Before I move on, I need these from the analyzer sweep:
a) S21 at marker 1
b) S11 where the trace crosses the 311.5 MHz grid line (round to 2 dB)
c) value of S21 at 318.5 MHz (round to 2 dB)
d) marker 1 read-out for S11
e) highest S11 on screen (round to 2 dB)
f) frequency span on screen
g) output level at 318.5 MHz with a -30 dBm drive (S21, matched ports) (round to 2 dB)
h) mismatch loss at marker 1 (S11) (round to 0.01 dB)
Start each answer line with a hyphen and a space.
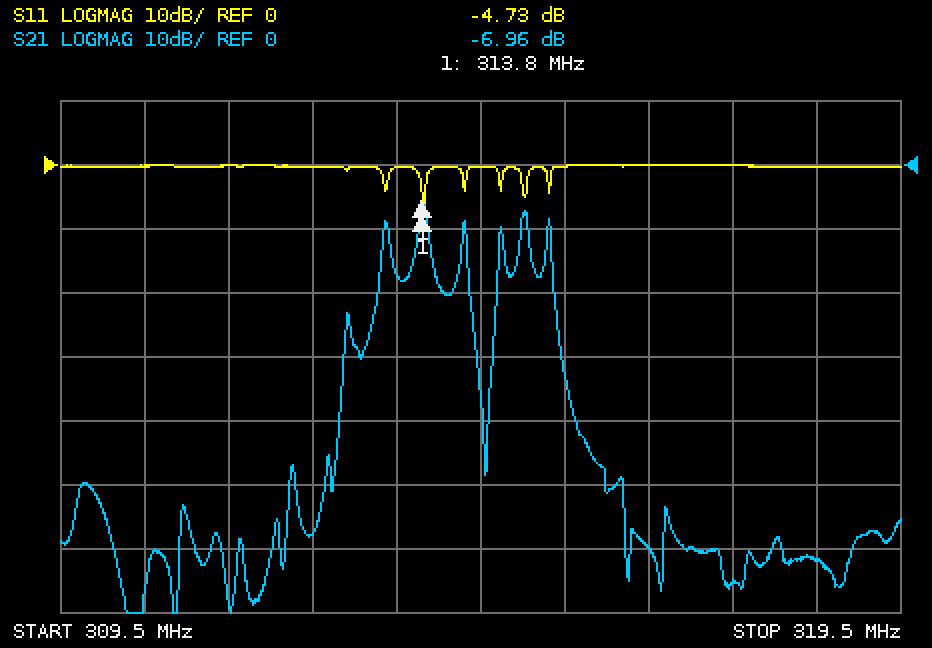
- -6.96 dB
- 0 dB
- -62 dB
- -4.73 dB
- 0 dB
- 10 MHz
- -92 dBm
- 1.78 dB
